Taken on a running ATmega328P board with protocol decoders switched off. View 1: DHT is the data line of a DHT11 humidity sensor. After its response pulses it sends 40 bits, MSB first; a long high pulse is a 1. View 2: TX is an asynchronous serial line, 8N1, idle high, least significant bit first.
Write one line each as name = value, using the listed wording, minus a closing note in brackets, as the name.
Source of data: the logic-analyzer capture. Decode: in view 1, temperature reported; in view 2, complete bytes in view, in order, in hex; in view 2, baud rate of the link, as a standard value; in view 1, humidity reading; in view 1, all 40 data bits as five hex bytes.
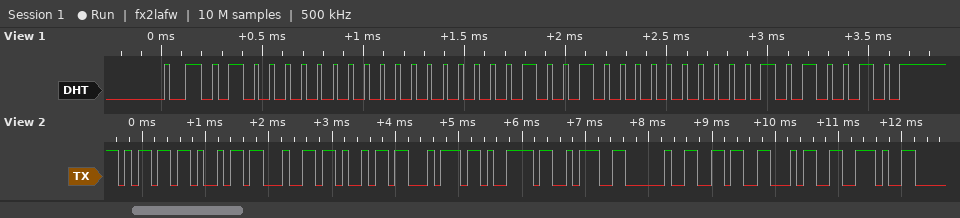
in view 1, temperature reported = 18.0 °C
in view 2, complete bytes in view, in order, in hex = 6D 69 64 69 74 79 3A 20 36 34 2E
in view 2, baud rate of the link, as a standard value = 9600 baud
in view 1, humidity reading = 64 %
in view 1, all 40 data bits as five hex bytes = 40 00 12 00 52
